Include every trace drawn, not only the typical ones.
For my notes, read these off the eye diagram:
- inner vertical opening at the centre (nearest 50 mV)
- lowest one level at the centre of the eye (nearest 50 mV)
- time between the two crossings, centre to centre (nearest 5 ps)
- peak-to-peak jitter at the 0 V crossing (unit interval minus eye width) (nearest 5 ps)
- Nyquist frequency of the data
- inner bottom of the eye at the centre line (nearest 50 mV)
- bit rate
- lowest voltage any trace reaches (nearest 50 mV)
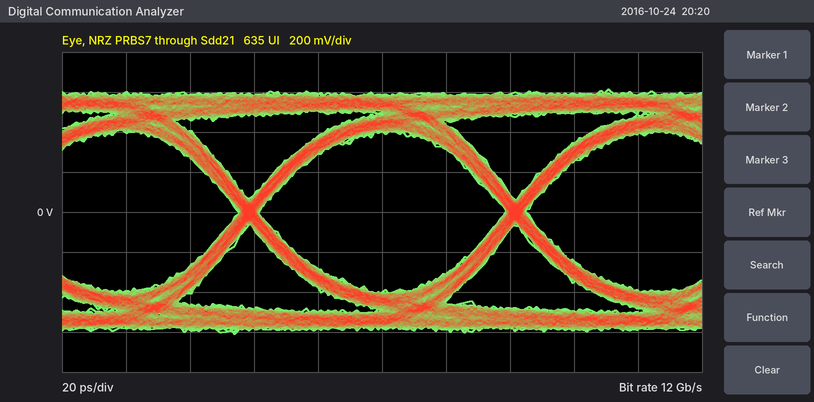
800 mV
400 mV
85 ps
5 ps
6 GHz
-400 mV
12 Gb/s
-600 mV
